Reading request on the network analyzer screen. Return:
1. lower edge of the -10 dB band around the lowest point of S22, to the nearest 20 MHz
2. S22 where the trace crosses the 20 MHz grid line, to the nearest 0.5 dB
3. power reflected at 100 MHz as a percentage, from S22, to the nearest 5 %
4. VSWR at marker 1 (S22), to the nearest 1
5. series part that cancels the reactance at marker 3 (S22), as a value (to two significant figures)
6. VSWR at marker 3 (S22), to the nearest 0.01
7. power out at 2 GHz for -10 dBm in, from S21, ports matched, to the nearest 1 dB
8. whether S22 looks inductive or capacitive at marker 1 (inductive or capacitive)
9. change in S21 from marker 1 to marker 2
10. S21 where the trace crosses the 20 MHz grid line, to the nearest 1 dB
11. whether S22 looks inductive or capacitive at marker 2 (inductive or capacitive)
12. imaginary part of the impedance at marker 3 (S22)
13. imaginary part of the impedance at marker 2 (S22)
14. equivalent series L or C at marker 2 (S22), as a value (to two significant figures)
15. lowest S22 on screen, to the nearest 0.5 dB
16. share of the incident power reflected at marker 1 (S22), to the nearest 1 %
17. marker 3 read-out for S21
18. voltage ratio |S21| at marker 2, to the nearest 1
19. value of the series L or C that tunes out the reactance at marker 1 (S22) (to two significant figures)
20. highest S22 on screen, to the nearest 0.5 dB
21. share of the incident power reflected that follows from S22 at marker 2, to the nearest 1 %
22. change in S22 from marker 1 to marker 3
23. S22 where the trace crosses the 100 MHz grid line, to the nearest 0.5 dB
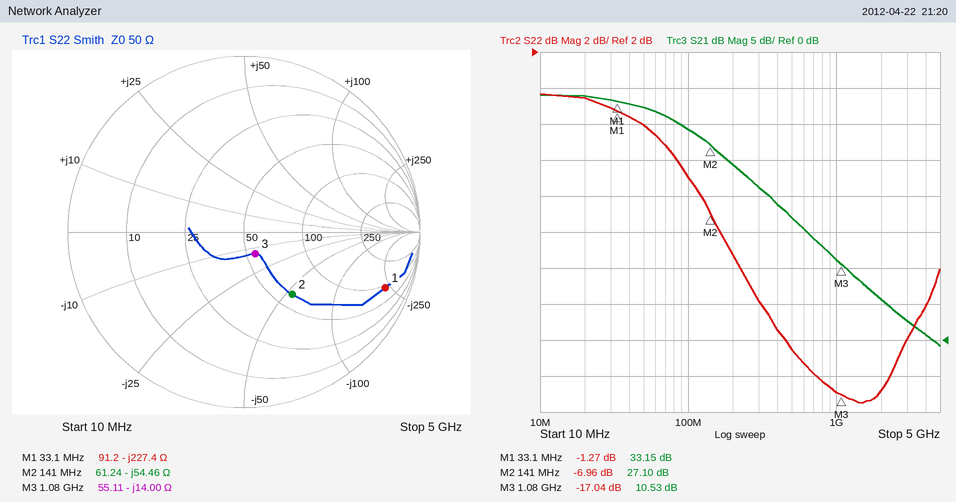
220 MHz
-0.5 dB
30 %
14
2.1 nH
1.33
-4 dBm
capacitive
-6.05 dB
34 dB
capacitive
-14.00 Ω
-54.46 Ω
21 pF
-17.5 dB
75 %
10.53 dB
23
1.1 µH
-0.5 dB
20 %
-15.77 dB
-5.0 dB
